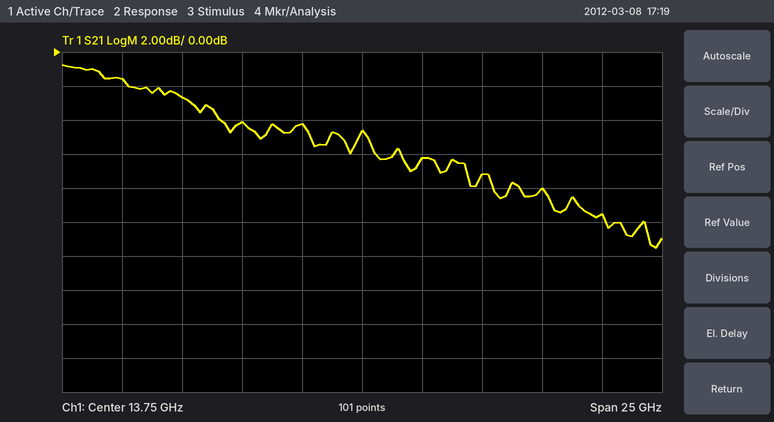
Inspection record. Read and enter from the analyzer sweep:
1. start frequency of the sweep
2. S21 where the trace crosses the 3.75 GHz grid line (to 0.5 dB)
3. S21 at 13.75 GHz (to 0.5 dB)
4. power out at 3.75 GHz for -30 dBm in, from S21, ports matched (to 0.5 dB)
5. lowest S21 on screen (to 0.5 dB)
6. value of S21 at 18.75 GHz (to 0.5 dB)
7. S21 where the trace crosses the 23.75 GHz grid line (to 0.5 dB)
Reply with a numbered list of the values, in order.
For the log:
1. 1.25 GHz
2. -1.5 dB
3. -4.5 dB
4. -31.5 dBm
5. -11.5 dB
6. -7.0 dB
7. -9.5 dB
